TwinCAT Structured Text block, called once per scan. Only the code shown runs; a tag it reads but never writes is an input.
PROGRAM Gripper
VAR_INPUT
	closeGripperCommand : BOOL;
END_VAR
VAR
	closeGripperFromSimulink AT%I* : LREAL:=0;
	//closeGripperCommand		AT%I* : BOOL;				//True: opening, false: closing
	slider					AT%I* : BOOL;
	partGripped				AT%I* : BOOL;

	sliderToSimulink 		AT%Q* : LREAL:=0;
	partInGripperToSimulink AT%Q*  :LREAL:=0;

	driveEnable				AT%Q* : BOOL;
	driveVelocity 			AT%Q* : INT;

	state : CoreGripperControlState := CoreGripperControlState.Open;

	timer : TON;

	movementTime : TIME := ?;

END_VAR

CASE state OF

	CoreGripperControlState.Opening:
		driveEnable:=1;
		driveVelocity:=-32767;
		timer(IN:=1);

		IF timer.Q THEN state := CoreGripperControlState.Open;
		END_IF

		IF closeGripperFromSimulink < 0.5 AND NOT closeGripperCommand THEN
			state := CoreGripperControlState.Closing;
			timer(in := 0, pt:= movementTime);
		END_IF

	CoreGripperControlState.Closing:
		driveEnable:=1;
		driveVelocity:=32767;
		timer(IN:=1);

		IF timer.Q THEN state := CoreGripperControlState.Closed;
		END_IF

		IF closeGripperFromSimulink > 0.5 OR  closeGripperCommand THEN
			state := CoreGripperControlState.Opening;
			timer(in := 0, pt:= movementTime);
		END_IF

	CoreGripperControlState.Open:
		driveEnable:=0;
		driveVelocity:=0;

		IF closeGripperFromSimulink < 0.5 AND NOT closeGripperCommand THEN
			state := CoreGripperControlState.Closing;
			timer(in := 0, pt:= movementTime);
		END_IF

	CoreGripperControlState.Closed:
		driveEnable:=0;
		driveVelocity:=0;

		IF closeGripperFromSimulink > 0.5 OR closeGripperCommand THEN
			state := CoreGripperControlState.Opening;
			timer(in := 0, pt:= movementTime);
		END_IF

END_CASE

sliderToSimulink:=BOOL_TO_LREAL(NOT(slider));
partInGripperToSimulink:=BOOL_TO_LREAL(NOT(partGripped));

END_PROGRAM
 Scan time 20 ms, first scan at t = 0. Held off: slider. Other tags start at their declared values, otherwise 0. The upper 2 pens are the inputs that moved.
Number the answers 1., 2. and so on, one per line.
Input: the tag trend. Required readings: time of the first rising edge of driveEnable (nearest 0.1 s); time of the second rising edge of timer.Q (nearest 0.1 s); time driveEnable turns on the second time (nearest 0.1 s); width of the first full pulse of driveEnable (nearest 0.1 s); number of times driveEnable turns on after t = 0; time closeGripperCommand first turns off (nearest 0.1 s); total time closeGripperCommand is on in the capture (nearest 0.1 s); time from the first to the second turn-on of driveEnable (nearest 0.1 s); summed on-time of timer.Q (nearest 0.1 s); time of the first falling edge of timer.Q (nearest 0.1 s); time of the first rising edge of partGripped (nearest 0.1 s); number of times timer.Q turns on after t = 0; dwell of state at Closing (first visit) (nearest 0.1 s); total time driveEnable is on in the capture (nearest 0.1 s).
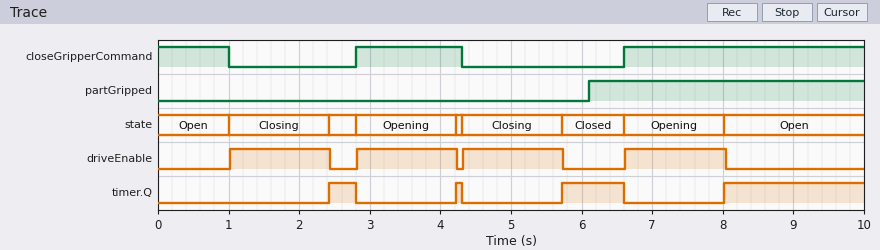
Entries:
1. 1.0 s
2. 4.2 s
3. 2.8 s
4. 1.4 s
5. 4
6. 1.0 s
7. 5.9 s
8. 1.8 s
9. 3.3 s
10. 2.8 s
11. 6.1 s
12. 4
13. 1.4 s
14. 5.7 s
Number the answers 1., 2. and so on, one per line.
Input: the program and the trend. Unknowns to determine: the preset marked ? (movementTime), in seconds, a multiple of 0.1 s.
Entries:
1. 1.4 s
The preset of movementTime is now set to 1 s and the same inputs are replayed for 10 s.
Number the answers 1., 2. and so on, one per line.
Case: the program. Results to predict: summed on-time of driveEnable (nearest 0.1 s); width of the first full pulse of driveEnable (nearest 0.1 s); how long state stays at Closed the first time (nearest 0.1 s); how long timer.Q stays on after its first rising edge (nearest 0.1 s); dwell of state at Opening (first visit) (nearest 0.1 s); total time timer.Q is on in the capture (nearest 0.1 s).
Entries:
1. 4.1 s
2. 1.0 s
3. 0.8 s
4. 0.8 s
5. 1.0 s
6. 4.9 s
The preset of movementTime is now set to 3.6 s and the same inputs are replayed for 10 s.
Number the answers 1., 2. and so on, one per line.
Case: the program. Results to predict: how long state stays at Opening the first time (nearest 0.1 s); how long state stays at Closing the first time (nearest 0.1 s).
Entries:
1. 1.5 s
2. 1.8 s
